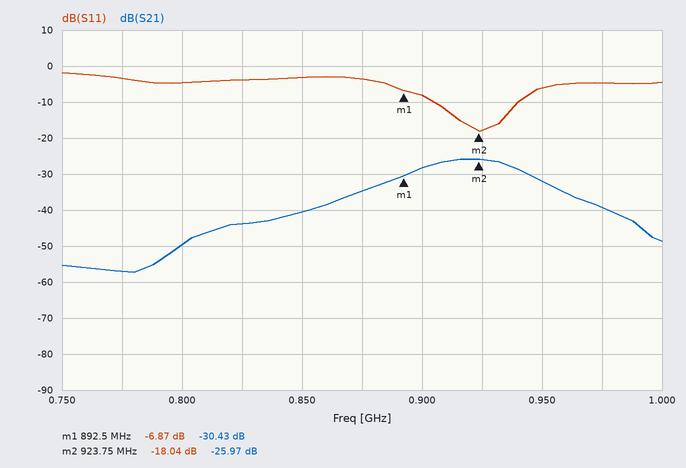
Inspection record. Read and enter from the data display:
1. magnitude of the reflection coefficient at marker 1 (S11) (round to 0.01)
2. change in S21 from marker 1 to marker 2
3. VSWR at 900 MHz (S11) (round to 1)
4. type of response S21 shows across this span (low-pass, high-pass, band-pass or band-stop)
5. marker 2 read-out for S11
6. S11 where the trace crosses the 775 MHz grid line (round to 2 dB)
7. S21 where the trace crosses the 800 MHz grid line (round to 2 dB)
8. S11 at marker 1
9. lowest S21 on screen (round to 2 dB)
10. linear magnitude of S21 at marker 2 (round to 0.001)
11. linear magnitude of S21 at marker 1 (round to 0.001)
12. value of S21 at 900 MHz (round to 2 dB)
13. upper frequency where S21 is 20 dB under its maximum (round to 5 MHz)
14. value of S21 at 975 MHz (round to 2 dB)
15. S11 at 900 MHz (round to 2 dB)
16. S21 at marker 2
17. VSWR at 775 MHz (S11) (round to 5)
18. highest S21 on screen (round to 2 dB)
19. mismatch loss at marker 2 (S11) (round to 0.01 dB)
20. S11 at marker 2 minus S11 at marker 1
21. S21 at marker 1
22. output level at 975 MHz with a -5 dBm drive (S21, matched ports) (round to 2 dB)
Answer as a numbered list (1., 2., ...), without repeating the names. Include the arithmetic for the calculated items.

1. 10^(-6.87/20) ≈ 0.45
2. -25.97 − (-30.43) = 4.46 dB
3. |Γ| = 10^(-8/20) = 0.3981; VSWR = (1 + 0.3981)/(1 − 0.3981) ≈ 2
4. band-pass
5. -18.04 dB
6. -4 dB
7. -50 dB
8. -6.87 dB
9. -58 dB
10. 10^(-25.97/20) ≈ 0.050
11. 10^(-30.43/20) ≈ 0.030
12. -28 dB
13. 995 MHz
14. -40 dB
15. -8 dB
16. -25.97 dB
17. |Γ| = 10^(-4/20) = 0.6310; VSWR = (1 + 0.6310)/(1 − 0.6310) ≈ 4.42, so 5 to the nearest 5
18. -26 dB
19. −10 log10(1 − 10^(-18.04/10)) ≈ 0.07 dB
20. -18.04 − (-6.87) = -11.17 dB
21. -30.43 dB
22. -5 dBm + (-40 dB) = -44 dBm
